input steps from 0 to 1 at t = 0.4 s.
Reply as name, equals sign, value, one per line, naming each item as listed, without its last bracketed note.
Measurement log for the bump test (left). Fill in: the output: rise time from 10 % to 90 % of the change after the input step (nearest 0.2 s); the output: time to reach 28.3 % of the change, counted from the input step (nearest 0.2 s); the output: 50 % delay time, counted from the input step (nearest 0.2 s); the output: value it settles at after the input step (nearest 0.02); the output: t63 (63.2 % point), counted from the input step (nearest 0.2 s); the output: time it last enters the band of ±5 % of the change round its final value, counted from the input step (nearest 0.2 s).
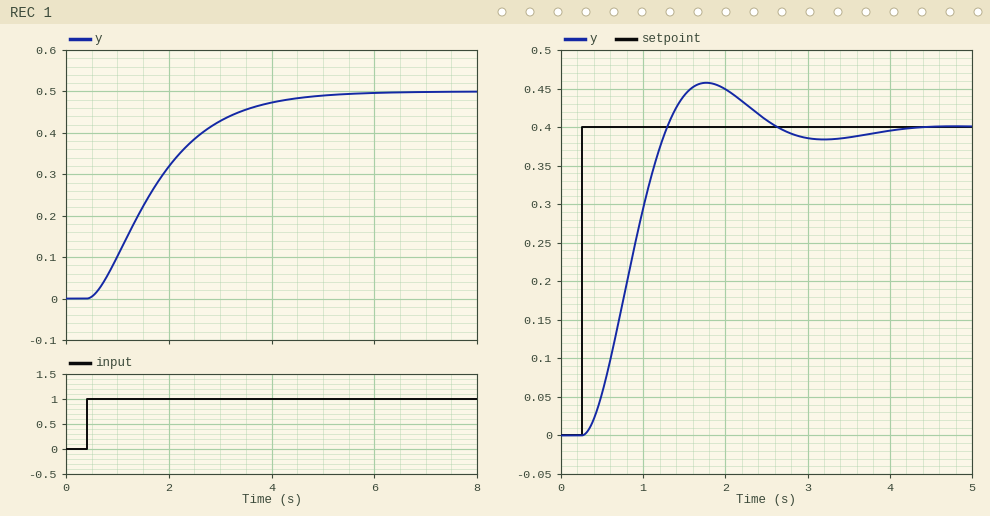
the output: rise time from 10 % to 90 % of the change after the input step = 2.6 s
the output: time to reach 28.3 % of the change, counted from the input step = 0.8 s
the output: 50 % delay time, counted from the input step = 1.2 s
the output: value it settles at after the input step = 0.50
the output: t63 (63.2 % point), counted from the input step = 1.6 s
the output: time it last enters the band of ±5 % of the change round its final value, counted from the input step = 3.6 s
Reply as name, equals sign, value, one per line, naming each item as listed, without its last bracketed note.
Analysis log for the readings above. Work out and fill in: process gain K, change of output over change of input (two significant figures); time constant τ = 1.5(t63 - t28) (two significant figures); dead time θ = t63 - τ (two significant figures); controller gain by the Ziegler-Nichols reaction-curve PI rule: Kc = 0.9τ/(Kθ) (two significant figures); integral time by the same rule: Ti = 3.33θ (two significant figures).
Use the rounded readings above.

process gain K, change of output over change of input = 0.50
time constant τ = 1.5(t63 - t28) = 1.2 s
dead time θ = t63 - τ = 0.40 s
controller gain by the Ziegler-Nichols reaction-curve PI rule: Kc = 0.9τ/(Kθ) = 5.4
integral time by the same rule: Ti = 3.33θ = 1.3 s
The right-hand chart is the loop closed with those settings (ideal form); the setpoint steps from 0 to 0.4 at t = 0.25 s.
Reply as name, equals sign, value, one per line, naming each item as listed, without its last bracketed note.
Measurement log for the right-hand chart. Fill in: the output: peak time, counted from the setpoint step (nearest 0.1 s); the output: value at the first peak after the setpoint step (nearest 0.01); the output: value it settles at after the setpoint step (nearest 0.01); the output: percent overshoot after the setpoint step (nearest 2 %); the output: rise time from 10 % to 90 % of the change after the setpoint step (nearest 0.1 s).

the output: peak time, counted from the setpoint step = 1.5 s
the output: value at the first peak after the setpoint step = 0.46
the output: value it settles at after the setpoint step = 0.40
the output: percent overshoot after the setpoint step = 14 %
the output: rise time from 10 % to 90 % of the change after the setpoint step = 0.7 s
